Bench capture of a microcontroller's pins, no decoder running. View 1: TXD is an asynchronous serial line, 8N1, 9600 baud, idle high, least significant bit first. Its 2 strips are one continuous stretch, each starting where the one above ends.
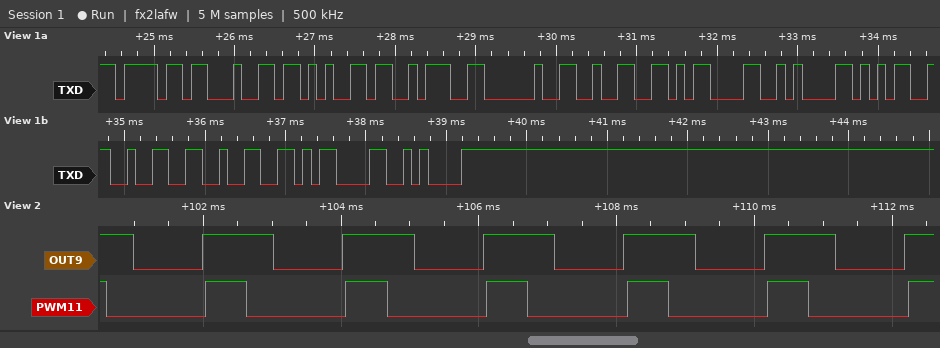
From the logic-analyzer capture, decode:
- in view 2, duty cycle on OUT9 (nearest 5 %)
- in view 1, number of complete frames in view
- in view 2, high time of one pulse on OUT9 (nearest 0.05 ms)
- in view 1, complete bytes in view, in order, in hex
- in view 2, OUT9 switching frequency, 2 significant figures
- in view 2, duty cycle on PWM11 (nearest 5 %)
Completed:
50 %
13
1.05 ms
6F 64 65 3A 20 32 0D 0A 35 32 32 0D 0A
490 Hz
30 %
